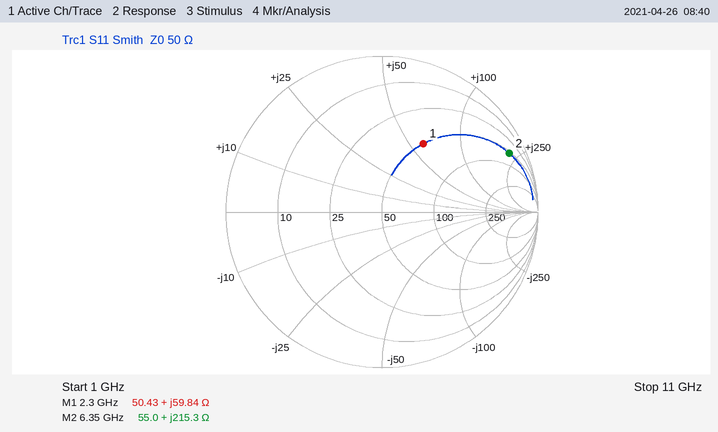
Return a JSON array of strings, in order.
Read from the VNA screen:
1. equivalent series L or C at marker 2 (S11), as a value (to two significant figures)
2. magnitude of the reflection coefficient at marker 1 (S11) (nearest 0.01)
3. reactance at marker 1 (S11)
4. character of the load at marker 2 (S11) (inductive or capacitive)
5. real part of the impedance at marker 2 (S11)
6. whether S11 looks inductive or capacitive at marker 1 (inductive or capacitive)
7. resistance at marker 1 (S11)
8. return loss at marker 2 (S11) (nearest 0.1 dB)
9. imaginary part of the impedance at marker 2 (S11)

["5.4 nH", "0.51", "+59.84 Ω", "inductive", "55.0 Ω", "inductive", "50.43 Ω", "0.9 dB", "+215.3 Ω"]
